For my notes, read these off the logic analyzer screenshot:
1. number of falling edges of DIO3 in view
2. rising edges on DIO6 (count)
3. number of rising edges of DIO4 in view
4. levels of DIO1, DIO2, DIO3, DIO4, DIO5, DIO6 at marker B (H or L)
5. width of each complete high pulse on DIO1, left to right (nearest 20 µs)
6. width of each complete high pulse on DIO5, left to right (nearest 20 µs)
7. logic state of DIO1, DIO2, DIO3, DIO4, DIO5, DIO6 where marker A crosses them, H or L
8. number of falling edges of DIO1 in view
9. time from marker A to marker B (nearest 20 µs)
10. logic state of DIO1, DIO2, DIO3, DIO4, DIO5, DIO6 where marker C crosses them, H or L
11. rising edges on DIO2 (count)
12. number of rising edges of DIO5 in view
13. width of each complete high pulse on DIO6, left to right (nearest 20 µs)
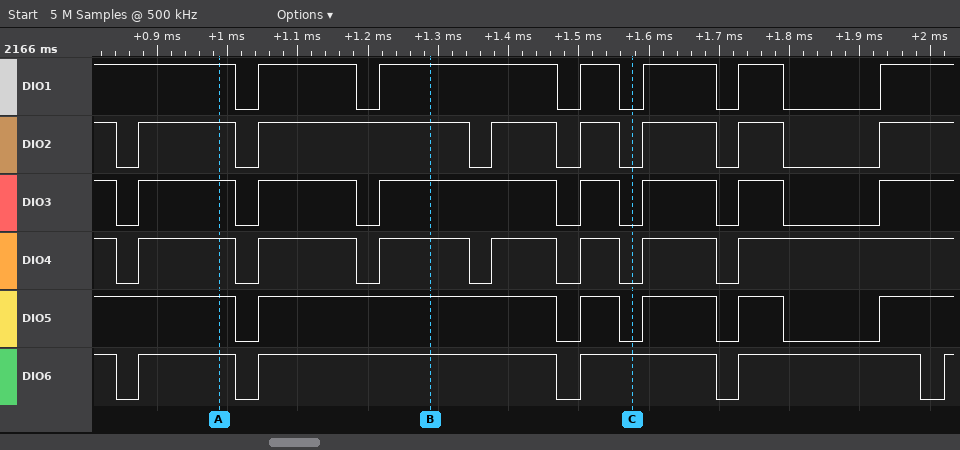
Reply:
7
5
7
DIO1=H, DIO2=H, DIO3=H, DIO4=H, DIO5=H, DIO6=H
140 µs, 260 µs, 60 µs, 100 µs, 60 µs
420 µs, 60 µs, 100 µs, 60 µs
DIO1=H, DIO2=H, DIO3=H, DIO4=H, DIO5=H, DIO6=H
6
300 µs
DIO1=L, DIO2=L, DIO3=L, DIO4=L, DIO5=L, DIO6=H
7
5
140 µs, 420 µs, 200 µs, 260 µs
